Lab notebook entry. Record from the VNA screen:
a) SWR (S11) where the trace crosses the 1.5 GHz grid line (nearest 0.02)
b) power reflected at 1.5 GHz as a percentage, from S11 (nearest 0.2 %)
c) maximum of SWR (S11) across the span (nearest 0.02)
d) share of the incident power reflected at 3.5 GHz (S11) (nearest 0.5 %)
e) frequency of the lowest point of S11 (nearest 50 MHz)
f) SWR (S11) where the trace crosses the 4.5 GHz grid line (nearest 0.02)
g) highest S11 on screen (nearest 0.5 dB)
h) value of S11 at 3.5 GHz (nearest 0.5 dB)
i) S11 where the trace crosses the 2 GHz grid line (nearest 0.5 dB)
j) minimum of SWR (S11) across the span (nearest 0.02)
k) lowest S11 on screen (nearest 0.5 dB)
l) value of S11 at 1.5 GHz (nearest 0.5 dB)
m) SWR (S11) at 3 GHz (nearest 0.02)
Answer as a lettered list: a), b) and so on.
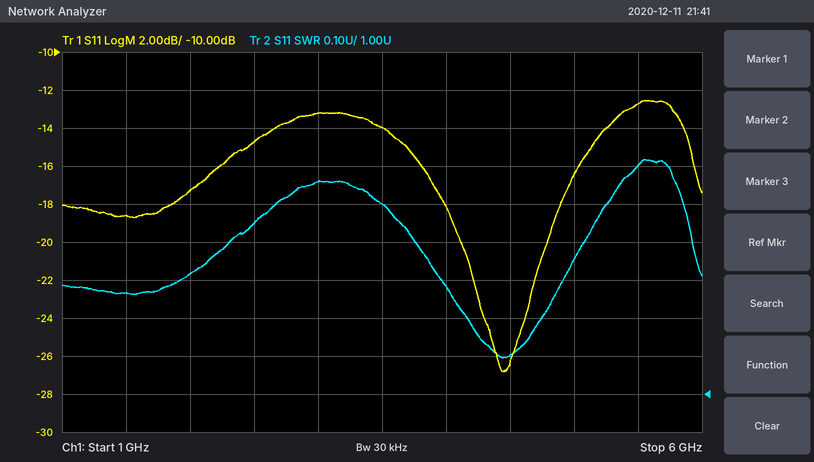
a) 1.26
b) 1.4 %
c) 1.62
d) 4.0 %
e) 4.45 GHz
f) 1.10
g) -12.5 dB
h) -14.0 dB
i) -17.5 dB
j) 1.10
k) -27.0 dB
l) -18.5 dB
m) 1.56
